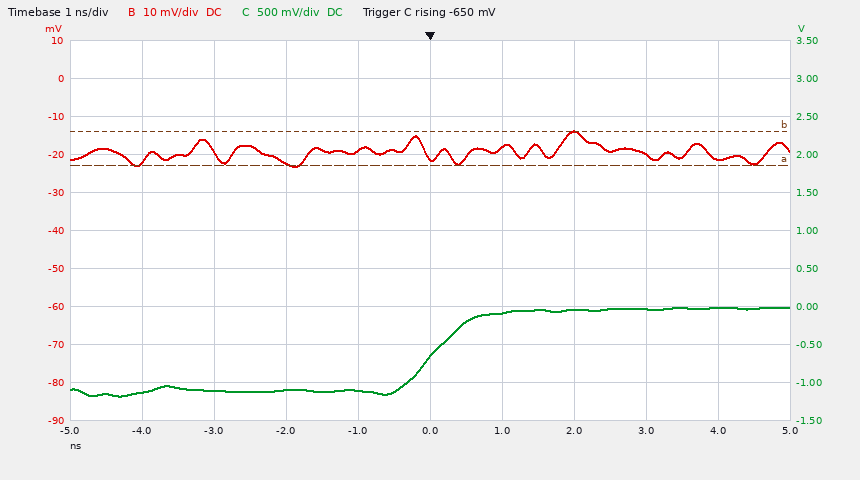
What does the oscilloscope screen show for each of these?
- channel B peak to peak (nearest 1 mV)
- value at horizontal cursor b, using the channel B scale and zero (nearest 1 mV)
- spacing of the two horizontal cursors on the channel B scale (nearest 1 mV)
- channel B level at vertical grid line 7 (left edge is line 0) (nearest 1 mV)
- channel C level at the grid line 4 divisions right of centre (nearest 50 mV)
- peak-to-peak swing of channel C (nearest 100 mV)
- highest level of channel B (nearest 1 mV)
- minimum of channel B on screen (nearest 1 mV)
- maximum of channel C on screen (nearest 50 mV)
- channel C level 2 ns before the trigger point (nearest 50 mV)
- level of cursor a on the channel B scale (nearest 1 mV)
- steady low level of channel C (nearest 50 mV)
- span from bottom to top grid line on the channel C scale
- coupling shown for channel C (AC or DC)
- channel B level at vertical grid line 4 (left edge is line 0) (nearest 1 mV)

9 mV
-14 mV
9 mV
-14 mV
0 mV
1.20 V
-14 mV
-23 mV
0 mV
-1.10 V
-23 mV
-1.10 V
5 V
DC
-19 mV
